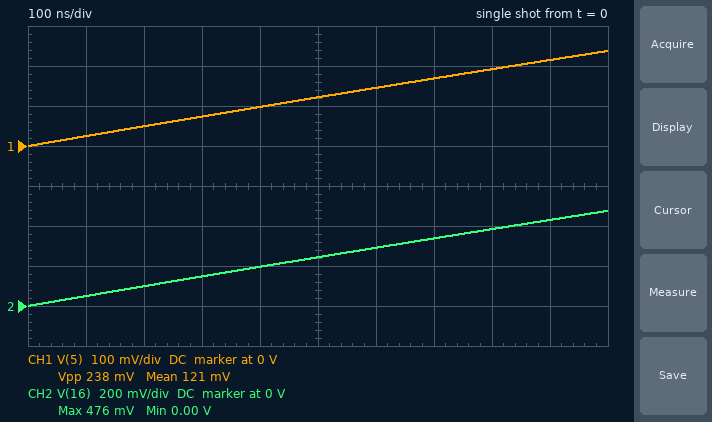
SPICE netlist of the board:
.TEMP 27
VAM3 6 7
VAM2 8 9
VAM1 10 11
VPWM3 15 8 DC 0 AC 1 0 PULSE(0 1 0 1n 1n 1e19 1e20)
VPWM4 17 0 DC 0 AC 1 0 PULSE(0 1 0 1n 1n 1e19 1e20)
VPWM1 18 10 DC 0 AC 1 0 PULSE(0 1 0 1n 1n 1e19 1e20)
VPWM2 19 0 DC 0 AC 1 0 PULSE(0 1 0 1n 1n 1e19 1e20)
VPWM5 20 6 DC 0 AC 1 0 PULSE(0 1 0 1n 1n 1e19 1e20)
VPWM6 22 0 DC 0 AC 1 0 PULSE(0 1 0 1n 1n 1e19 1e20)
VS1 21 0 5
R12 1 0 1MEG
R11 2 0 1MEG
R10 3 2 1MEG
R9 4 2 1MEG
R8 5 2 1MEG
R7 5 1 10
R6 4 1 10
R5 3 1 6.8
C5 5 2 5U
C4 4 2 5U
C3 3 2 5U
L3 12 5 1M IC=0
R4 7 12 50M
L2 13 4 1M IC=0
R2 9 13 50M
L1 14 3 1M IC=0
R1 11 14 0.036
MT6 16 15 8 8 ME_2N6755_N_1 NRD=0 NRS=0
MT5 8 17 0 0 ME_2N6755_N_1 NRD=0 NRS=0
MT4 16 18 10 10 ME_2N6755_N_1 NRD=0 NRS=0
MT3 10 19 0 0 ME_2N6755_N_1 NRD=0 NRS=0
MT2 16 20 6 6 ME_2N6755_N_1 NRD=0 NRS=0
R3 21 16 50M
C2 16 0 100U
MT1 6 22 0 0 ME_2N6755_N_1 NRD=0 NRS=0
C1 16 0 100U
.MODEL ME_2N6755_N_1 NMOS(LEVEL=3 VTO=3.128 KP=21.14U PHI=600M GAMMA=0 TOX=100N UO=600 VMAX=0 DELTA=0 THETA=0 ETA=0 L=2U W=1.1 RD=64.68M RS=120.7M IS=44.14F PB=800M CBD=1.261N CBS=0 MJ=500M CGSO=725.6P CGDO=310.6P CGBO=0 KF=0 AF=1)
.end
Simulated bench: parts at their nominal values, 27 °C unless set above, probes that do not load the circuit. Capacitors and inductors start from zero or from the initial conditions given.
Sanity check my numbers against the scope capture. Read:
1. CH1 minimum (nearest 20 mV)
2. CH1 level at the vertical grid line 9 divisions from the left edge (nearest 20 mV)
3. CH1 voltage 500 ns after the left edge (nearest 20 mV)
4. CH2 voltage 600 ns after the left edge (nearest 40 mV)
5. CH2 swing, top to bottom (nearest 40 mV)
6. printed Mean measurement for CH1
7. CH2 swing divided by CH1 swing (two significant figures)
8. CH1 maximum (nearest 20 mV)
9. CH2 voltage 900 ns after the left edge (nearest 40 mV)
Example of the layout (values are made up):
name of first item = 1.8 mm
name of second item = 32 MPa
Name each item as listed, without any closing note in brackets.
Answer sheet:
CH1 minimum = 0 V
CH1 level at the vertical grid line 9 divisions from the left edge = 220 mV
CH1 voltage 500 ns after the left edge = 120 mV
CH2 voltage 600 ns after the left edge = 280 mV
CH2 swing, top to bottom = 480 mV
printed Mean measurement for CH1 = 121 mV
CH2 swing divided by CH1 swing = 2.0
CH1 maximum = 240 mV
CH2 voltage 900 ns after the left edge = 440 mV
